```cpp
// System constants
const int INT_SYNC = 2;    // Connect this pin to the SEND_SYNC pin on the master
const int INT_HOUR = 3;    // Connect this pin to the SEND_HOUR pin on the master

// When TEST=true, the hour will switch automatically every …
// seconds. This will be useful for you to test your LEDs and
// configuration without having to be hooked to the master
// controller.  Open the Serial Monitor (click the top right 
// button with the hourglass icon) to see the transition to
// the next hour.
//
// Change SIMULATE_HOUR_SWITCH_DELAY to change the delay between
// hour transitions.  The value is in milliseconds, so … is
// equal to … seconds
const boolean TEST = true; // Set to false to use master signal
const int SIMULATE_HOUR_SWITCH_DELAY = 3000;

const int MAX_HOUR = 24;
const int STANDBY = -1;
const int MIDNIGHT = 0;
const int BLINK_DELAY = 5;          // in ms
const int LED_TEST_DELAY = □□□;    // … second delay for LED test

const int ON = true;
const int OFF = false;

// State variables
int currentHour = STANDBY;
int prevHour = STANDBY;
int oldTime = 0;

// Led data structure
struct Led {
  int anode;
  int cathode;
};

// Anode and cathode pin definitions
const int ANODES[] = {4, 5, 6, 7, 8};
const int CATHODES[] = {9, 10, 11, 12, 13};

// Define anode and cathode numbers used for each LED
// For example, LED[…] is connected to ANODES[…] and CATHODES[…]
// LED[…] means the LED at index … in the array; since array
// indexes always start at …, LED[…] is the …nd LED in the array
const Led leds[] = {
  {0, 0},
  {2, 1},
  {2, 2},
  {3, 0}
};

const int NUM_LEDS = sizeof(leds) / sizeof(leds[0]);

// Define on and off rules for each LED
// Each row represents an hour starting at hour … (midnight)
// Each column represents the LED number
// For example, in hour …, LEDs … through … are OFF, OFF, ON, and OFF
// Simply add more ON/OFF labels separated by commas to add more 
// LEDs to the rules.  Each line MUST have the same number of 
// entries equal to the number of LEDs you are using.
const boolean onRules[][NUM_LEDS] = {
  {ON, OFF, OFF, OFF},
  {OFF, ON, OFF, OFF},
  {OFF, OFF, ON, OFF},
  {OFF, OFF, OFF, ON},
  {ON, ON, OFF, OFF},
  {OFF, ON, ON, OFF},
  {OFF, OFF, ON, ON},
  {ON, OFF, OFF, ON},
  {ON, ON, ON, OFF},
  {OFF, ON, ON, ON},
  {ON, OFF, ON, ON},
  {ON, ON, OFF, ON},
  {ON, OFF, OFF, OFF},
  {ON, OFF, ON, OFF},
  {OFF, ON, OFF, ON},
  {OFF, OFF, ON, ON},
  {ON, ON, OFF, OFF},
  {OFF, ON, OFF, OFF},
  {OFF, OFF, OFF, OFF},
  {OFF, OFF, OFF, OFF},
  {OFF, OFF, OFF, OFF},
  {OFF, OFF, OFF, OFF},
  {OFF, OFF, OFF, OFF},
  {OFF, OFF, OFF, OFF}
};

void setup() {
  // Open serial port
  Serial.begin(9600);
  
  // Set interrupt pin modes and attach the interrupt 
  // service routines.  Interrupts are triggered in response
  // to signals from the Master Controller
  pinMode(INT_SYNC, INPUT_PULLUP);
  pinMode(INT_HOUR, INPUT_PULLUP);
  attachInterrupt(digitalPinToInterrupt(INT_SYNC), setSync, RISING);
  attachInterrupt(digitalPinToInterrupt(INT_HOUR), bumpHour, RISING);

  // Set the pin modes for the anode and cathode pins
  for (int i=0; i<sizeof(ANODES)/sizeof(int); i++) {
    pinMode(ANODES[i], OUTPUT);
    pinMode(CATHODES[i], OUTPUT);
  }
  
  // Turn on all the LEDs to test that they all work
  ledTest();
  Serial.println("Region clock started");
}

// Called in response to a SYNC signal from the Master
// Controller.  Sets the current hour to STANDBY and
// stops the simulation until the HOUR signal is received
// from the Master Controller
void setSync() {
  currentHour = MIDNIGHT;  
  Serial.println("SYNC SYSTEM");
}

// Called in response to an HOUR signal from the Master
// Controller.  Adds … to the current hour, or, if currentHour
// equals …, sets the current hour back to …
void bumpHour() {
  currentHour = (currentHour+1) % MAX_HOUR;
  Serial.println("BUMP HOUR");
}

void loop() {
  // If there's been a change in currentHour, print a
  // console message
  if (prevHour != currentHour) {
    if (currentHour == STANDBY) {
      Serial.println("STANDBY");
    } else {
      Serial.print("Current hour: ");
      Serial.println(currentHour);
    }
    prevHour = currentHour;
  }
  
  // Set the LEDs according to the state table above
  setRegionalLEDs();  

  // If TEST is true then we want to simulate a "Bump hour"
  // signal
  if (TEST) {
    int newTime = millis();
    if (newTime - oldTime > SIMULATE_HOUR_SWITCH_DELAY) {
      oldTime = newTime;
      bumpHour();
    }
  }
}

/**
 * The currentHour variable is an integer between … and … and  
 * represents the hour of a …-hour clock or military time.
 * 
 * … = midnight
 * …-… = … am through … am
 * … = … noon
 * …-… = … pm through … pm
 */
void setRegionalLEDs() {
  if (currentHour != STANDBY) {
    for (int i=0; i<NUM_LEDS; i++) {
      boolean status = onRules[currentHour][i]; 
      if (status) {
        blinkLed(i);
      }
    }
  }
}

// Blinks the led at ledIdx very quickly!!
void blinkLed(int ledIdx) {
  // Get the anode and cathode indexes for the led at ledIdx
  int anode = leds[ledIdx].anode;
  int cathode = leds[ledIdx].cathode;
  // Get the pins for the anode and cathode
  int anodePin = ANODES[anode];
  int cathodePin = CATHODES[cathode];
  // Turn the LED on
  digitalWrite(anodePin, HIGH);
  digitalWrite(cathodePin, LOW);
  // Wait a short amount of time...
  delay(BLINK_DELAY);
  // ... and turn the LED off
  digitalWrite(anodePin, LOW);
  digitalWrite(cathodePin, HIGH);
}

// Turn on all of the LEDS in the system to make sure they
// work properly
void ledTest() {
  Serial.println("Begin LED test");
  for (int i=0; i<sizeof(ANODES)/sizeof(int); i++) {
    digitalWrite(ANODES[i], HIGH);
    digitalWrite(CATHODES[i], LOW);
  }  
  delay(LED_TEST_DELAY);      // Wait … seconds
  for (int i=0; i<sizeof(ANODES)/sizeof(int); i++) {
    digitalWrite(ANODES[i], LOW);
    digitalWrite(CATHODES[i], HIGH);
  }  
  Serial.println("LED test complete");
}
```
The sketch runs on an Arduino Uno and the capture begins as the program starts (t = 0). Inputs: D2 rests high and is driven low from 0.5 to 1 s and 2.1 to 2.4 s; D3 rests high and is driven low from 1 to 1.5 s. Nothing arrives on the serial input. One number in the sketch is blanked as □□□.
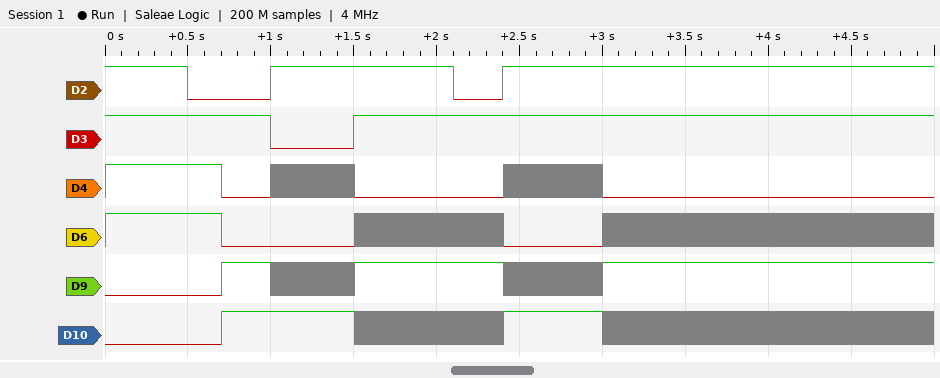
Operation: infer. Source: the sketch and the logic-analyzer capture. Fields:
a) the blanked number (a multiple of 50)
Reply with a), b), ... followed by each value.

a) 700
